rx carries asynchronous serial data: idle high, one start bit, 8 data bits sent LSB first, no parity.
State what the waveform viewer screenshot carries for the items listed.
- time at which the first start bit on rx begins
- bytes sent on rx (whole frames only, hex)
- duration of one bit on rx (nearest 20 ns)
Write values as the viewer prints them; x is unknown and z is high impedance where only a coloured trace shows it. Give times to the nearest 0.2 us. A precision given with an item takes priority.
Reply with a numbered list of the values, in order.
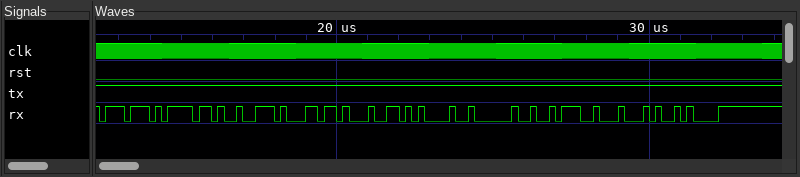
1. 12.4 us
2. 77, 6F, 72, 6C, 64, 21, 20, 3A, 44, 0A
3. 200 ns
